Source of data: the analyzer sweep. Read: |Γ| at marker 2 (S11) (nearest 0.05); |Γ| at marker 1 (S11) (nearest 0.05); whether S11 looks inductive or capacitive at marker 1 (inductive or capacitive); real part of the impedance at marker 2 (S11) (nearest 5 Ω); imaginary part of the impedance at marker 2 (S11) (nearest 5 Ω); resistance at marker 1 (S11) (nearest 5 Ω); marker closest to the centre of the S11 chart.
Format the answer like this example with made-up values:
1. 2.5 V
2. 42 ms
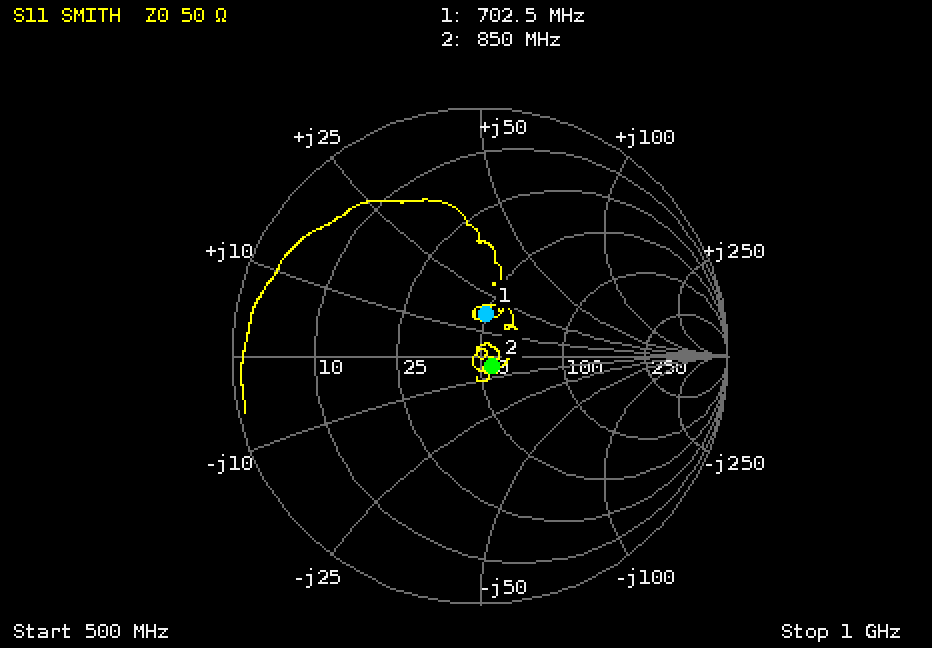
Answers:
1. 0.05
2. 0.15
3. inductive
4. 55 Ω
5. -5 Ω
6. 50 Ω
7. marker 2
